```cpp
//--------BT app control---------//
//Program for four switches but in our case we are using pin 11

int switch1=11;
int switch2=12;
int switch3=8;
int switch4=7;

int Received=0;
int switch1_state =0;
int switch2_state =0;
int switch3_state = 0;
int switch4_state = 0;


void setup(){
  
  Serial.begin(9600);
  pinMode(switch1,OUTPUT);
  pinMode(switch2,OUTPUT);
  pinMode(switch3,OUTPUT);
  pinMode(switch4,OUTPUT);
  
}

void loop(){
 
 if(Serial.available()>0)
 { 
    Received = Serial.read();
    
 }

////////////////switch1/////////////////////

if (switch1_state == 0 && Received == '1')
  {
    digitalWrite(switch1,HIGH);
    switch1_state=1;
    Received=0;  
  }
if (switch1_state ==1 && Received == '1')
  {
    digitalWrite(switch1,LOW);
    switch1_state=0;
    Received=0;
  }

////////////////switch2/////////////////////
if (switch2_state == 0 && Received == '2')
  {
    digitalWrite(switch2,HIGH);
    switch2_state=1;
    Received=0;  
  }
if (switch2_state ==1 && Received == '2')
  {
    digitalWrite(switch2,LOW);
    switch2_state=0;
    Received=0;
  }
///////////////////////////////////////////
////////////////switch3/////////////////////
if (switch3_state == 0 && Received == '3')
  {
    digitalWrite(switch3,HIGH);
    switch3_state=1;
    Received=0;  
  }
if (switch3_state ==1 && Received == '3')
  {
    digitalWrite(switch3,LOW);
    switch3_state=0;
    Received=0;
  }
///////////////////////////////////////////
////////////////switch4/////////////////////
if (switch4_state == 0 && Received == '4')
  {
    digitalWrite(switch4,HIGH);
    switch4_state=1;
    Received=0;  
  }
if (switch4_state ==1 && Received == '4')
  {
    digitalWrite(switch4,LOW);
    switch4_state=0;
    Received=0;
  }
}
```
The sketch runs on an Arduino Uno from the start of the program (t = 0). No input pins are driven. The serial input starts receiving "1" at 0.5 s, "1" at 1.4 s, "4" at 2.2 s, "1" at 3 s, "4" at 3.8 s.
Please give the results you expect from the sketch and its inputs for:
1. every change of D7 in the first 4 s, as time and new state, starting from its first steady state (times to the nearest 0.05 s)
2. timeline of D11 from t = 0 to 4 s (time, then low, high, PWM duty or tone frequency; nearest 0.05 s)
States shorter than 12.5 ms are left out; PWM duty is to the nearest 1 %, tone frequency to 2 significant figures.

0 s low; 2.2 s high; 3.8 s low
0 s low; 0.5 s high; 1.4 s low; 3 s high
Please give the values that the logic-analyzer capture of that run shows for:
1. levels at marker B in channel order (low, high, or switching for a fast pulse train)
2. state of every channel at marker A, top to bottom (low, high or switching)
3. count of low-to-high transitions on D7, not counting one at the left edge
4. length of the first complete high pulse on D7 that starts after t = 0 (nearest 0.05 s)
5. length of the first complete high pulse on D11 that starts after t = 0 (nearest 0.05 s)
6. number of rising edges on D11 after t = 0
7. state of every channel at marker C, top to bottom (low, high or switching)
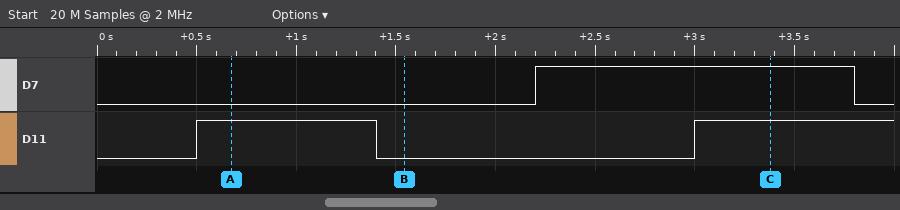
D7 low, D11 low
D7 low, D11 high
1
1.60 s
0.90 s
2
D7 high, D11 high
